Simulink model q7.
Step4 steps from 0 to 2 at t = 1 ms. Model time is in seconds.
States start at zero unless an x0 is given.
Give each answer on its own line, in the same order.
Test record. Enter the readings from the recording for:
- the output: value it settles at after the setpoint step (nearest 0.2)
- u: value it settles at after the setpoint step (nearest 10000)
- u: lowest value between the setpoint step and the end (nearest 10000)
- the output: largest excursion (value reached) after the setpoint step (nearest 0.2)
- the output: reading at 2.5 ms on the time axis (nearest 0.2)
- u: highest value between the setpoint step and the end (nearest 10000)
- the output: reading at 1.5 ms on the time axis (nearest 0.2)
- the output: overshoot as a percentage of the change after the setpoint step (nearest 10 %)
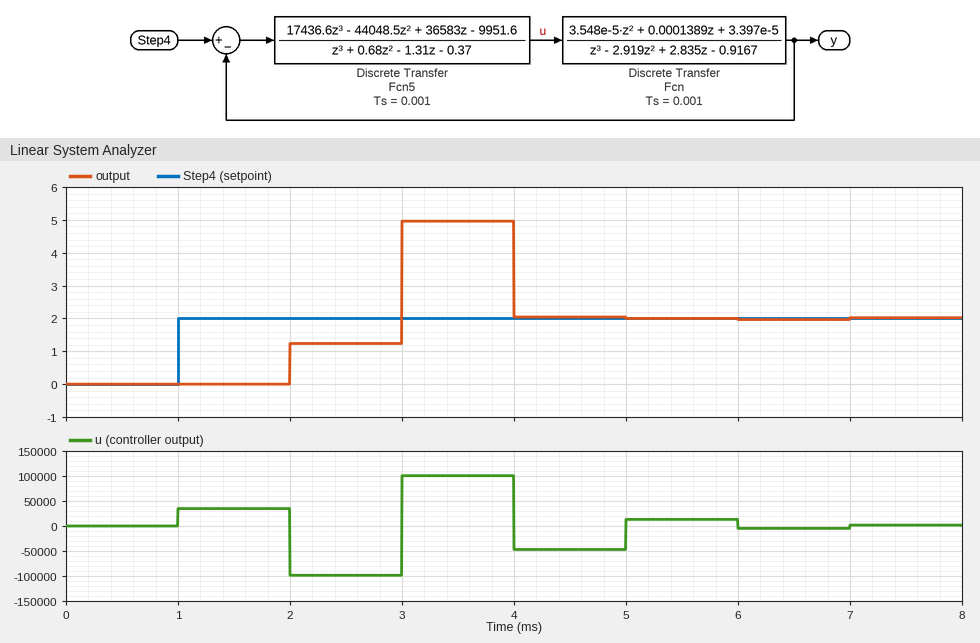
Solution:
2.0
0
-100000
5.0
1.2
100000
0.0
150 %
